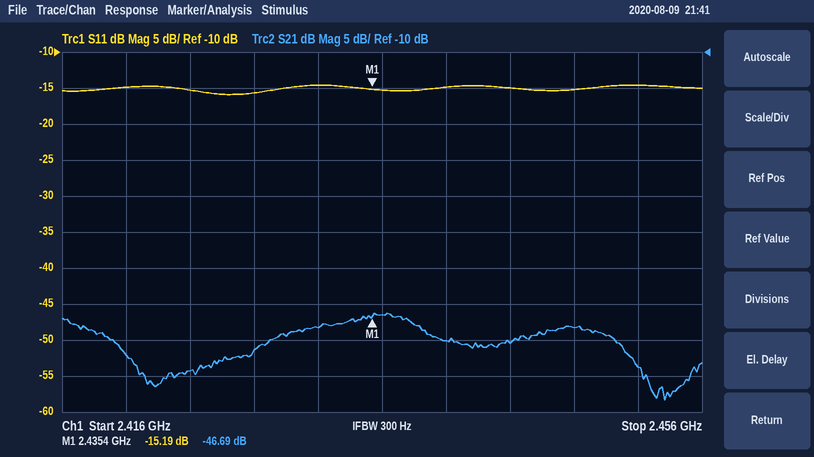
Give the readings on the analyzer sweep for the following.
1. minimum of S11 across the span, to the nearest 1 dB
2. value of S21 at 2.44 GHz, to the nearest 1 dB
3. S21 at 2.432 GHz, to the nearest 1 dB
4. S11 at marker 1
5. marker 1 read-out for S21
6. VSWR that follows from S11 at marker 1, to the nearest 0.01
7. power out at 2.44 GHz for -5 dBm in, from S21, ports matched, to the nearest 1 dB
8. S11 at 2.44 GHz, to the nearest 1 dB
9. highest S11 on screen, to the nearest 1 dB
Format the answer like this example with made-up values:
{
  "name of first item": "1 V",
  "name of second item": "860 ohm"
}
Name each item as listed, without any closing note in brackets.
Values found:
{
  "minimum of S11 across the span, to the nearest 1 dB": "-16 dB",
  "value of S21 at 2.44 GHz, to the nearest 1 dB": "-50 dB",
  "S21 at 2.432 GHz, to the nearest 1 dB": "-48 dB",
  "S11 at marker 1": "-15.19 dB",
  "marker 1 read-out for S21": "-46.69 dB",
  "VSWR that follows from S11 at marker 1, to the nearest 0.01": "1.42",
  "power out at 2.44 GHz for -5 dBm in, from S21, ports matched, to the nearest 1 dB": "-55 dBm",
  "S11 at 2.44 GHz, to the nearest 1 dB": "-15 dB",
  "highest S11 on screen, to the nearest 1 dB": "-15 dB"
}
